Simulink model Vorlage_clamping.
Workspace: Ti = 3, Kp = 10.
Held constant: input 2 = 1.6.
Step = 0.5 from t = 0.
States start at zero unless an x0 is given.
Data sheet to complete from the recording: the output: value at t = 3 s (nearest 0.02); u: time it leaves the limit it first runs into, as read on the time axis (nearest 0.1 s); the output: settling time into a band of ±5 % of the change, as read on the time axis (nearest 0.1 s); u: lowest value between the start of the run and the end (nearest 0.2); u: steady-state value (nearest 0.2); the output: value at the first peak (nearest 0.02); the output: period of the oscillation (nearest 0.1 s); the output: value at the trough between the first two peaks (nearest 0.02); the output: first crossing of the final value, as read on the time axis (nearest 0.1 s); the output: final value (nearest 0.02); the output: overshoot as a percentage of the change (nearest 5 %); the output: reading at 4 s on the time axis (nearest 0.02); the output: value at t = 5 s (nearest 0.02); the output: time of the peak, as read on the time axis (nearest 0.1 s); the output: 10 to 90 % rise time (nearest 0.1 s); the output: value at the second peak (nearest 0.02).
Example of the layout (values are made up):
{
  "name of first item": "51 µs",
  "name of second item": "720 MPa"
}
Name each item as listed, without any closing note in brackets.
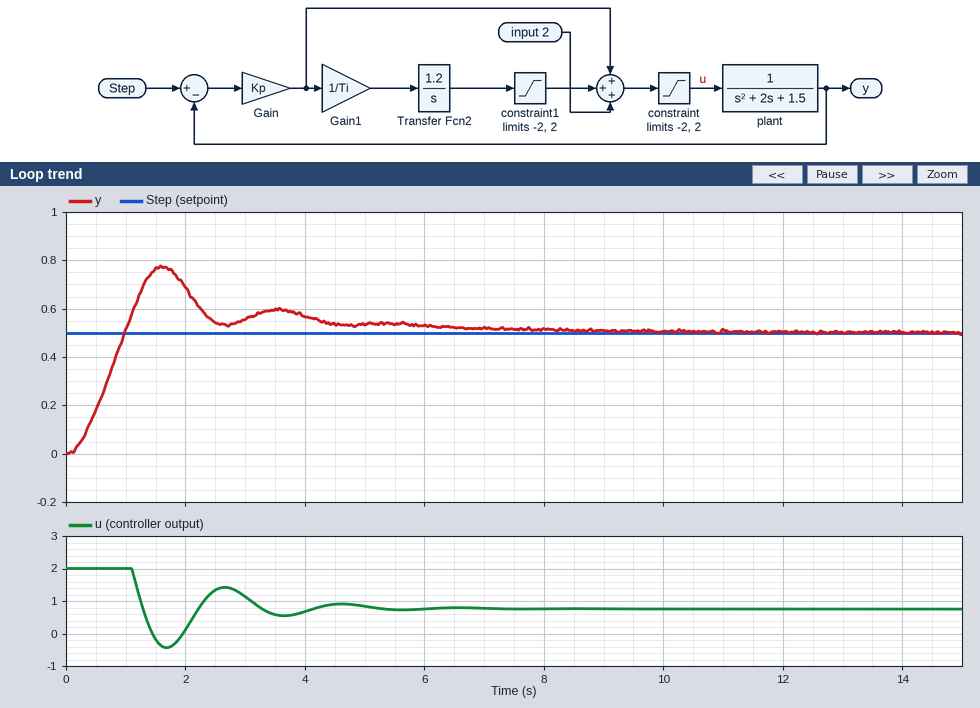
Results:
{
  "the output: value at t = 3 s": "0.56",
  "u: time it leaves the limit it first runs into, as read on the time axis": "1.1 s",
  "the output: settling time into a band of ±5 % of the change, as read on the time axis": "6.2 s",
  "u: lowest value between the start of the run and the end": "-0.4",
  "u: steady-state value": "0.8",
  "the output: value at the first peak": "0.78",
  "the output: period of the oscillation": "1.9 s",
  "the output: value at the trough between the first two peaks": "0.54",
  "the output: first crossing of the final value, as read on the time axis": "1.0 s",
  "the output: final value": "0.50",
  "the output: overshoot as a percentage of the change": "55 %",
  "the output: reading at 4 s on the time axis": "0.56",
  "the output: value at t = 5 s": "0.54",
  "the output: time of the peak, as read on the time axis": "1.6 s",
  "the output: 10 to 90 % rise time": "0.7 s",
  "the output: value at the second peak": "0.60"
}
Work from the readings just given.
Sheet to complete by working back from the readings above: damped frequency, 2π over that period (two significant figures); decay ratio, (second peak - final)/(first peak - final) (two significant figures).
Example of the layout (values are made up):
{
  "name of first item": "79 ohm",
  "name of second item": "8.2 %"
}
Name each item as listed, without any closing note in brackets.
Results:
{
  "damped frequency, 2π over that period": "3.3 rad/s",
  "decay ratio, (second peak - final)/(first peak - final)": "0.36"
}
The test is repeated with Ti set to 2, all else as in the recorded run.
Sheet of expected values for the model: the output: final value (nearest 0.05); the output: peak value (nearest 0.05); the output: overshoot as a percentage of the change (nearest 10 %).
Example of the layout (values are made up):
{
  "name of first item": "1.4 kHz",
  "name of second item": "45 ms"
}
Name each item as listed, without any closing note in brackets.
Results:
{
  "the output: final value": "0.50",
  "the output: peak value": "0.80",
  "the output: overshoot as a percentage of the change": "60 %"
}
